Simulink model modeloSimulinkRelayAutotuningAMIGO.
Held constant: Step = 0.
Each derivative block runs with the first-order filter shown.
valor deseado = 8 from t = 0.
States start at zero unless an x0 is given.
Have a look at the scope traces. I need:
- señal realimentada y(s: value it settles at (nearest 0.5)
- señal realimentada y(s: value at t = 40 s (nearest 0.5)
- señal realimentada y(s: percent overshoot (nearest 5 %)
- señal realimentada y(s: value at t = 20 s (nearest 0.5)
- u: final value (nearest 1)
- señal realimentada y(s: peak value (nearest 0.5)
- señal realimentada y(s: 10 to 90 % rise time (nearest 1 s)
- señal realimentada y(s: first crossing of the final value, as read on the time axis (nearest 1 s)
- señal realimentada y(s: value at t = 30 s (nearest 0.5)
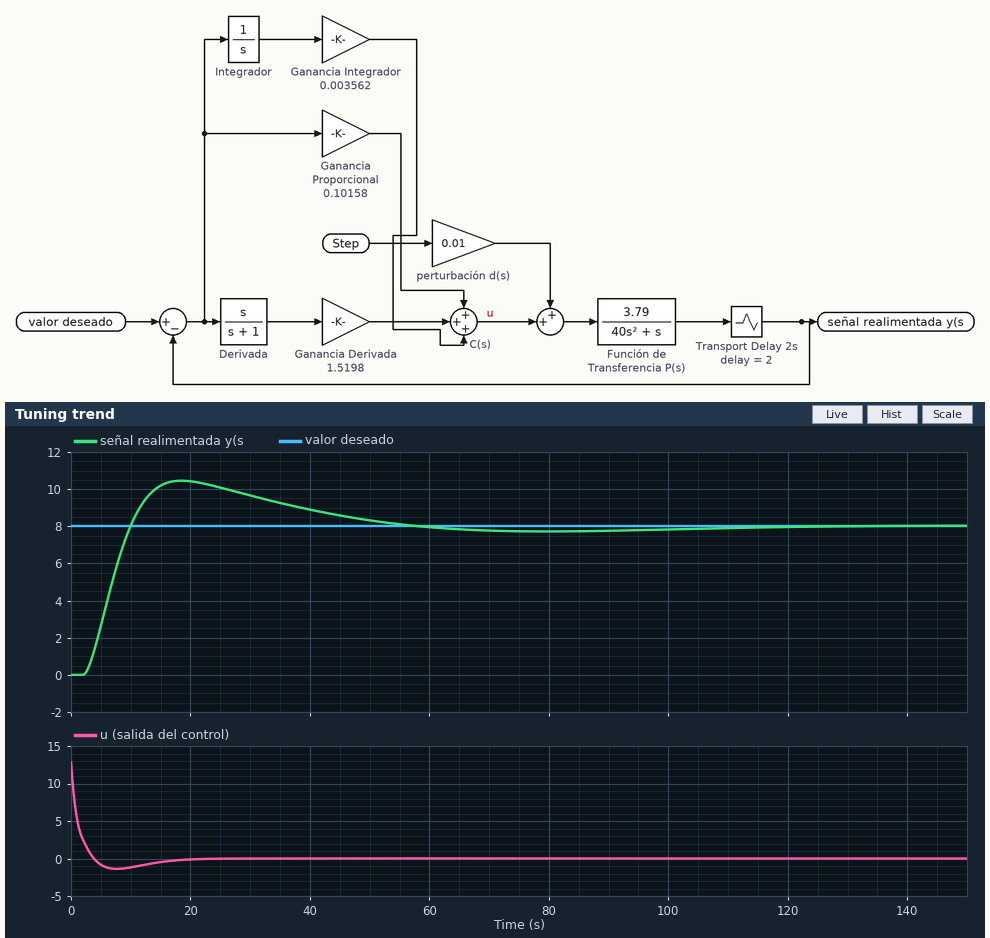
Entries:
8.0
9.0
30 %
10.5
0
10.5
6 s
10 s
9.5
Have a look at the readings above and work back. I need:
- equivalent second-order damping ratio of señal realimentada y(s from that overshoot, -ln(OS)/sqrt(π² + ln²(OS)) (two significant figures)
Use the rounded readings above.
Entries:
0.36
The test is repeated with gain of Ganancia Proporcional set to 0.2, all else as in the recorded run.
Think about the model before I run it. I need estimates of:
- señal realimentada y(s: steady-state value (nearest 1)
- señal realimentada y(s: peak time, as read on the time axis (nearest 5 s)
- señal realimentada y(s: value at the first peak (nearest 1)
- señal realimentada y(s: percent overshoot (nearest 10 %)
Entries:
8
15 s
12
50 %
